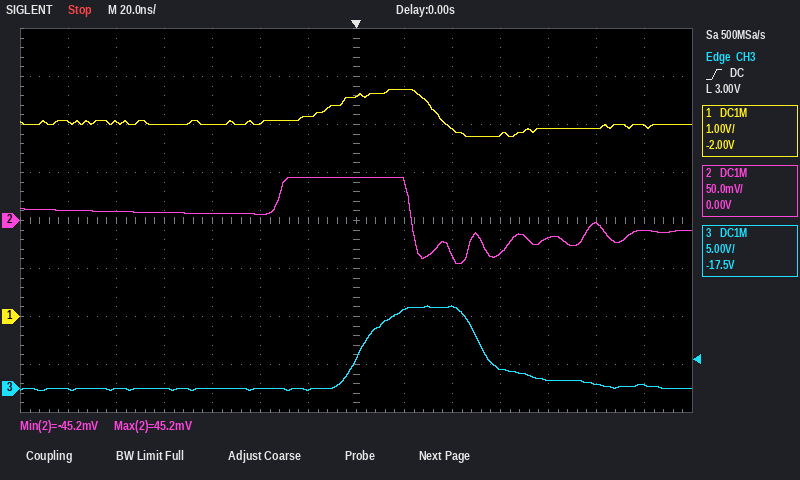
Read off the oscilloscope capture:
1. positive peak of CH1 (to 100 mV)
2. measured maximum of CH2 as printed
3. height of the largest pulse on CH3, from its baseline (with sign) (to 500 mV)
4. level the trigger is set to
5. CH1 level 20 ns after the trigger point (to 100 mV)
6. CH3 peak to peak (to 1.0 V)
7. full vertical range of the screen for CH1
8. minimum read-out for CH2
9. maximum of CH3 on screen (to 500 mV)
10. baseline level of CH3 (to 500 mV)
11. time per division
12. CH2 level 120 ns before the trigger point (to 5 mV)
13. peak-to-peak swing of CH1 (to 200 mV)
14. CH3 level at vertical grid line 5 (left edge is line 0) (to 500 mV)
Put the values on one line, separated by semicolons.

4.7 V; 45.2 mV; +8.5 V; 3.00 V; 4.7 V; 9.0 V; 8 V; -45.2 mV; 8.5 V; 0.0 V; 20 ns; 10 mV; 1.0 V; 0.0 V
